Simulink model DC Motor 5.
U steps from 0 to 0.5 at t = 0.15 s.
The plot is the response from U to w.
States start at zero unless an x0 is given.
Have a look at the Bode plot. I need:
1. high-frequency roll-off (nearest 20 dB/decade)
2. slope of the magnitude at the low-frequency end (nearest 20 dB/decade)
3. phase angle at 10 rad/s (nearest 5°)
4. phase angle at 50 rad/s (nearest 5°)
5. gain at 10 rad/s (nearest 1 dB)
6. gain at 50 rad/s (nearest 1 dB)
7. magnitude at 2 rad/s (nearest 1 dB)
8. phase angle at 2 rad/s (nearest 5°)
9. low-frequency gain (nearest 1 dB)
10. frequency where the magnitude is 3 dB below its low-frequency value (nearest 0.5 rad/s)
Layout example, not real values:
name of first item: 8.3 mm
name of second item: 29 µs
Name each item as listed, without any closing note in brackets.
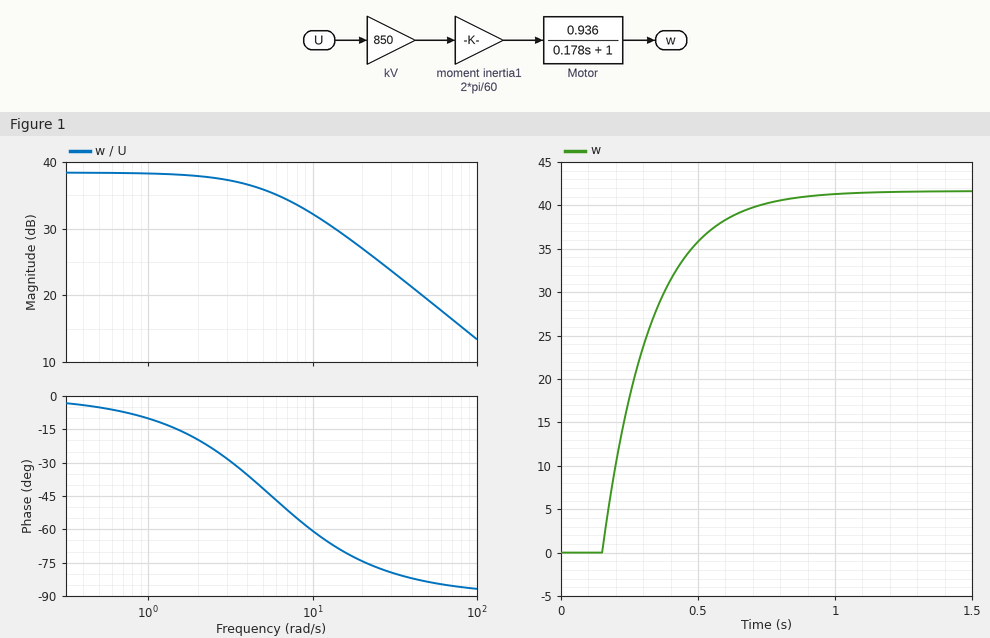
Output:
high-frequency roll-off: -20 dB/decade
slope of the magnitude at the low-frequency end: 0 dB/decade
phase angle at 10 rad/s: -60°
phase angle at 50 rad/s: -85°
gain at 10 rad/s: 32 dB
gain at 50 rad/s: 19 dB
magnitude at 2 rad/s: 38 dB
phase angle at 2 rad/s: -20°
low-frequency gain: 38 dB
frequency where the magnitude is 3 dB below its low-frequency value: 5.5 rad/s
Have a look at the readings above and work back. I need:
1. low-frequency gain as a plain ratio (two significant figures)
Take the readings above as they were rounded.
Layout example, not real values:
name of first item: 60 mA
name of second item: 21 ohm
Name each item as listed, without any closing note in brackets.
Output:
low-frequency gain as a plain ratio: 79
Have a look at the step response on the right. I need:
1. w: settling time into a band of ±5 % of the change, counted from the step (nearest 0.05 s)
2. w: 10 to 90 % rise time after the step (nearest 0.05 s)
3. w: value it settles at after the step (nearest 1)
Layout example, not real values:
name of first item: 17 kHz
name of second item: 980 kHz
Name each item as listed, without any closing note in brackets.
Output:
w: settling time into a band of ±5 % of the change, counted from the step: 0.55 s
w: 10 to 90 % rise time after the step: 0.40 s
w: value it settles at after the step: 42
